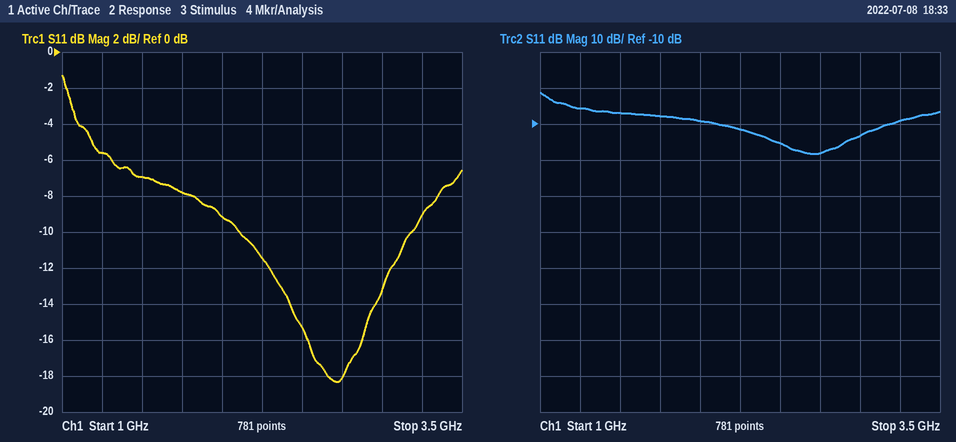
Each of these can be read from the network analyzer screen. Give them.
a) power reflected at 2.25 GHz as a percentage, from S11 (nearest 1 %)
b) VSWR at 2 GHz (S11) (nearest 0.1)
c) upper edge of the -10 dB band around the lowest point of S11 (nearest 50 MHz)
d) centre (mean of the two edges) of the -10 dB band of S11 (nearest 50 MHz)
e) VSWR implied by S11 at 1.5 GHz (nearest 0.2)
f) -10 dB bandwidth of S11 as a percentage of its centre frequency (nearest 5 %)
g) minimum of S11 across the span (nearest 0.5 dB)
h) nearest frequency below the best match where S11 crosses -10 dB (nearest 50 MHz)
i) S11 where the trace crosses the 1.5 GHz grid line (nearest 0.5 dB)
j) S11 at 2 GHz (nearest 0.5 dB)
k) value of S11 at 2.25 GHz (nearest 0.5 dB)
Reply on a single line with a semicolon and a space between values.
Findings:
7 %; 2.1; 3.20 GHz; 2.65 GHz; 2.6; 40 %; -18.5 dB; 2.10 GHz; -7.0 dB; -9.0 dB; -11.5 dB
